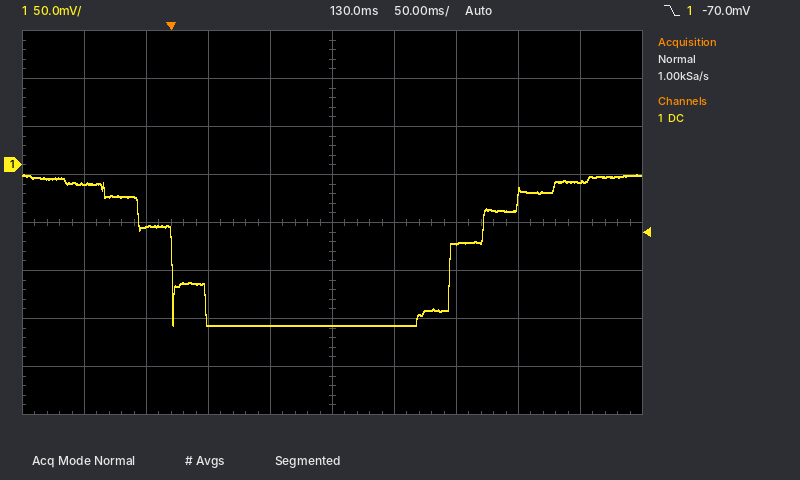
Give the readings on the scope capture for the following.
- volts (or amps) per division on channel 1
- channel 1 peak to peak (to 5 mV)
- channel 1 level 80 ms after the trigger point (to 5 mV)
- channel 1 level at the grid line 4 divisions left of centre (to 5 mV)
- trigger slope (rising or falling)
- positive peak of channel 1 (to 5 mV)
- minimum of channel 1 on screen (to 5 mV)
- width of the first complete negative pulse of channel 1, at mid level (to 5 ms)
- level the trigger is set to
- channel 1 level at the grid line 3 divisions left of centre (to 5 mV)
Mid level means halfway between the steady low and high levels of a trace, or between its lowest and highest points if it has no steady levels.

50 mV
155 mV
-165 mV
-20 mV
falling
-10 mV
-165 mV
225 ms
-70.0 mV
-65 mV
